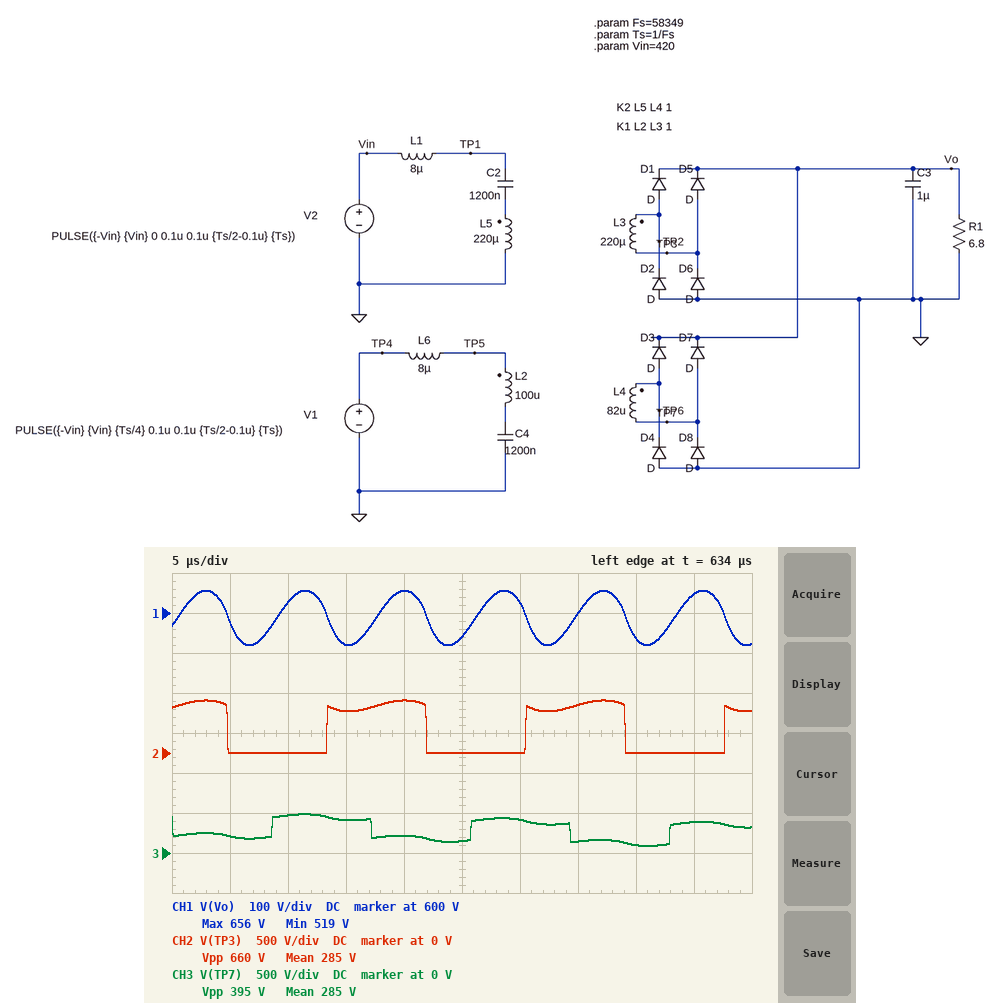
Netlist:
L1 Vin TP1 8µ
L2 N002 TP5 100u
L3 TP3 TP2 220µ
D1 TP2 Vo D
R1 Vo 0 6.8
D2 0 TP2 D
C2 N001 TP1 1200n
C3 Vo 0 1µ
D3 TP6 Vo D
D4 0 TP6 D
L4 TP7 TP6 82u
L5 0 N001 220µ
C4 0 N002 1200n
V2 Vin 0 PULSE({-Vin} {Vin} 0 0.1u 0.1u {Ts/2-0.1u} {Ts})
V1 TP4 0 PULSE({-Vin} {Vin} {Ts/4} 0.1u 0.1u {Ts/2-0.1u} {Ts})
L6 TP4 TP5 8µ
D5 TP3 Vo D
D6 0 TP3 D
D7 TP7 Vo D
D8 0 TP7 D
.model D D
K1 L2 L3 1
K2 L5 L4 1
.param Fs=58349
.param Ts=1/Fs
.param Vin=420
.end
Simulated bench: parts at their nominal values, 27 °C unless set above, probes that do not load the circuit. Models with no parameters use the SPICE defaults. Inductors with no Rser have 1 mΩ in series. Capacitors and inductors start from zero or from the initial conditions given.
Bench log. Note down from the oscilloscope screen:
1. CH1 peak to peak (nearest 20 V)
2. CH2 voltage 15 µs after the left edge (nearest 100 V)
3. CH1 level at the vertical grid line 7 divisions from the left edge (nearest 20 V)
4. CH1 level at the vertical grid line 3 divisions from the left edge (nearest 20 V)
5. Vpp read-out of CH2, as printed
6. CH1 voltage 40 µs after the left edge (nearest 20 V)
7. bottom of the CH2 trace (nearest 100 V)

140 V
500 V
600 V
520 V
660 V
540 V
0 V
